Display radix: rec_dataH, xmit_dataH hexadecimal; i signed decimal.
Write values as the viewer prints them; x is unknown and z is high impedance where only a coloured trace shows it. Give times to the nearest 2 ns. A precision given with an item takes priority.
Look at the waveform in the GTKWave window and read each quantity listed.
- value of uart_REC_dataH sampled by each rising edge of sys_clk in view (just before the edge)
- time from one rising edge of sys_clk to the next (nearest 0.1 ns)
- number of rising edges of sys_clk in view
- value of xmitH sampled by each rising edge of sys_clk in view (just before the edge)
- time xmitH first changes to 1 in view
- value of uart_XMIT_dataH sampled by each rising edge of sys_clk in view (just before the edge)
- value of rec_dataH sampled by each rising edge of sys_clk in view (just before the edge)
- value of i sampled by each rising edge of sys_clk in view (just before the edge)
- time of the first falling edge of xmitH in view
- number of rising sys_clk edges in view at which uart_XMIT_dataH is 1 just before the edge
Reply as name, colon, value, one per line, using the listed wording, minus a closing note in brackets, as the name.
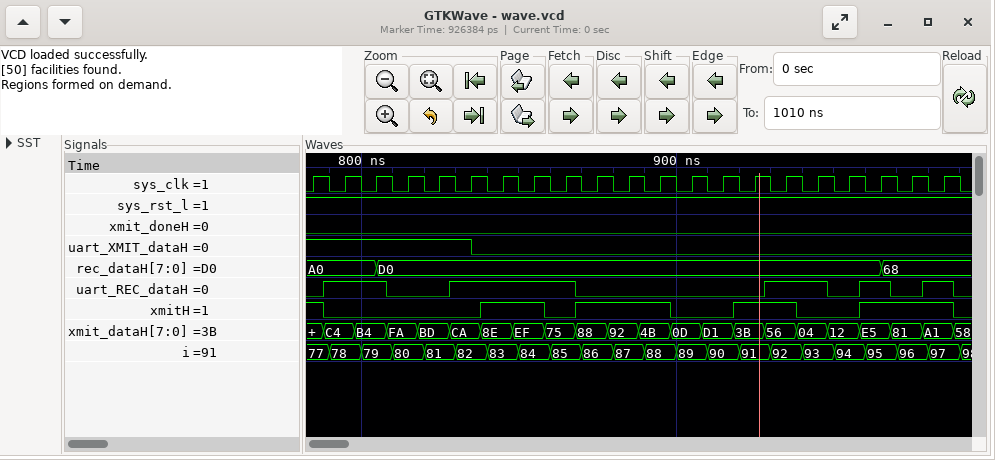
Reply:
value of uart_REC_dataH sampled by each rising edge of sys_clk in view: 0 1 1 0 0 1 1 1 1 0 0 0 0 0 0 1 1 0 1 0 1
time from one rising edge of sys_clk to the next: 10 ns
number of rising edges of sys_clk in view: 21
value of xmitH sampled by each rising edge of sys_clk in view: 1 0 0 0 0 0 1 1 0 1 1 1 0 0 1 1 0 0 1 1 1
time xmitH first changes to 1 in view: 838 ns
value of uart_XMIT_dataH sampled by each rising edge of sys_clk in view: 1 1 1 1 1 1 0 0 0 0 0 0 0 0 0 0 0 0 0 0 0
value of rec_dataH sampled by each rising edge of sys_clk in view: A0, A0, A0, D0, D0, D0, D0, D0, D0, D0, D0, D0, D0, D0, D0, D0, D0, D0, D0, 68, 68
value of i sampled by each rising edge of sys_clk in view: 77, 78, 79, 80, 81, 82, 83, 84, 85, 86, 87, 88, 89, 90, 91, 92, 93, 94, 95, 96, 97
time of the first falling edge of xmitH in view: 788 ns
number of rising sys_clk edges in view at which uart_XMIT_dataH is 1 just before the edge: 6
